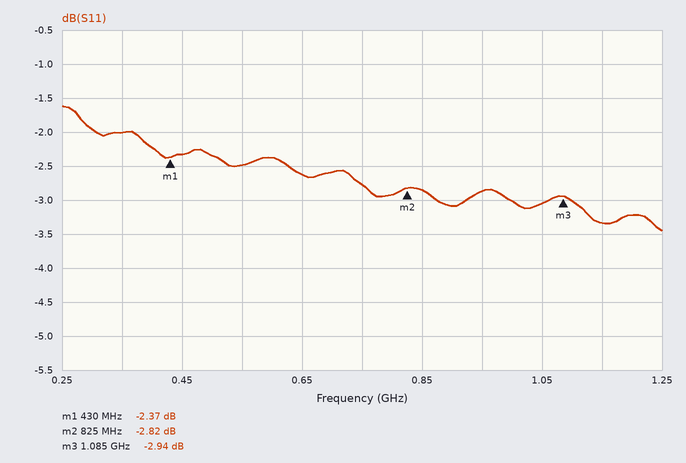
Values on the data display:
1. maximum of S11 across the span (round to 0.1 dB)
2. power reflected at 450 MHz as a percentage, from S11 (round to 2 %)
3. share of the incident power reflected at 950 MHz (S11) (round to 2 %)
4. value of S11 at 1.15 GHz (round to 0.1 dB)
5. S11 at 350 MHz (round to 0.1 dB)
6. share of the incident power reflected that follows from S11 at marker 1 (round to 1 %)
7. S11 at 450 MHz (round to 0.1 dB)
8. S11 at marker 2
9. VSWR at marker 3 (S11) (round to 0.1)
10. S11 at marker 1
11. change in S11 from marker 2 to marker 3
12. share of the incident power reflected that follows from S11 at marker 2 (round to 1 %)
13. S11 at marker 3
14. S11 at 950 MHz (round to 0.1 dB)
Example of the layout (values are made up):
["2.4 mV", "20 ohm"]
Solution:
["-1.6 dB", "58 %", "52 %", "-3.3 dB", "-2.0 dB", "58 %", "-2.3 dB", "-2.82 dB", "6.0", "-2.37 dB", "-0.12 dB", "52 %", "-2.94 dB", "-2.9 dB"]
